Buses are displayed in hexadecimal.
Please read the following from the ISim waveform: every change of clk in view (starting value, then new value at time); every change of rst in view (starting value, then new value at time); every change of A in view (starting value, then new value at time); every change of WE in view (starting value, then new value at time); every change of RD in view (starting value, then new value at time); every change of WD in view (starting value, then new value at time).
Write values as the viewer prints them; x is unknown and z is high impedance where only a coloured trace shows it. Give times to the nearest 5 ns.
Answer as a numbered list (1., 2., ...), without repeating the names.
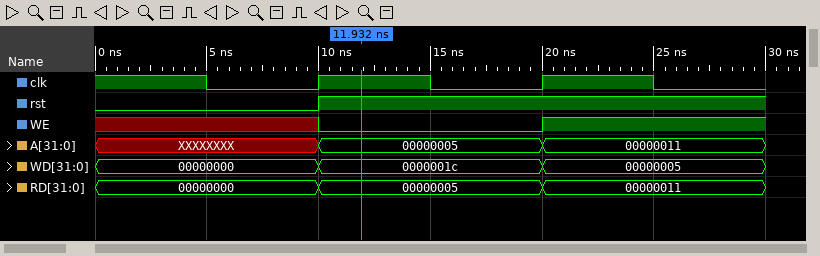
1. 1, 0 at 5 ns, 1 at 10 ns, 0 at 15 ns, 1 at 20 ns, 0 at 25 ns
2. 0, 1 at 10 ns
3. XXXXXXXX, 00000005 at 10 ns, 00000011 at 20 ns
4. x, 0 at 10 ns, 1 at 20 ns
5. 00000000, 00000005 at 10 ns, 00000011 at 20 ns
6. 00000000, 0000001c at 10 ns, 00000005 at 20 ns
